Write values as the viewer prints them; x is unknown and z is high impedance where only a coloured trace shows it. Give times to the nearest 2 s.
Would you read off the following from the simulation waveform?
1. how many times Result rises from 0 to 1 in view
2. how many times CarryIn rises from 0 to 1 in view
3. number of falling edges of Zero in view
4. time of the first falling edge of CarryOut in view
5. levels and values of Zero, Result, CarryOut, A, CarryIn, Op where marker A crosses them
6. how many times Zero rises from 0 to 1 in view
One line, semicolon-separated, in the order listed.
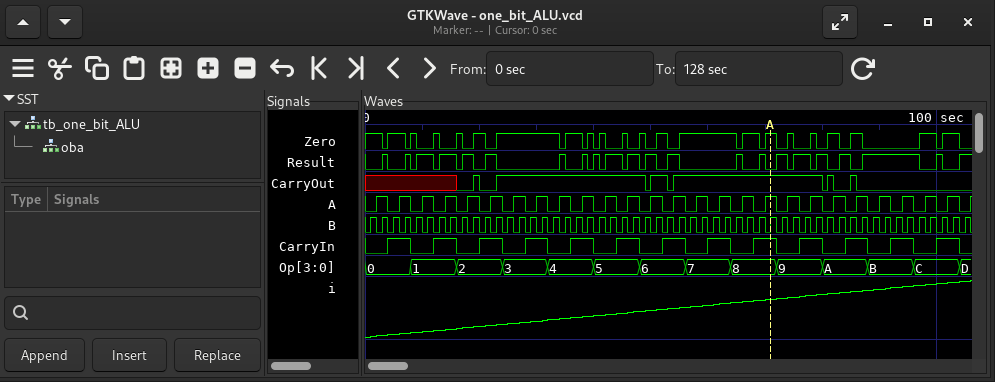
22; 13; 22; 20 s; Zero=1, Result=0, CarryOut=1, A=1, CarryIn=1, Op=8; 21
